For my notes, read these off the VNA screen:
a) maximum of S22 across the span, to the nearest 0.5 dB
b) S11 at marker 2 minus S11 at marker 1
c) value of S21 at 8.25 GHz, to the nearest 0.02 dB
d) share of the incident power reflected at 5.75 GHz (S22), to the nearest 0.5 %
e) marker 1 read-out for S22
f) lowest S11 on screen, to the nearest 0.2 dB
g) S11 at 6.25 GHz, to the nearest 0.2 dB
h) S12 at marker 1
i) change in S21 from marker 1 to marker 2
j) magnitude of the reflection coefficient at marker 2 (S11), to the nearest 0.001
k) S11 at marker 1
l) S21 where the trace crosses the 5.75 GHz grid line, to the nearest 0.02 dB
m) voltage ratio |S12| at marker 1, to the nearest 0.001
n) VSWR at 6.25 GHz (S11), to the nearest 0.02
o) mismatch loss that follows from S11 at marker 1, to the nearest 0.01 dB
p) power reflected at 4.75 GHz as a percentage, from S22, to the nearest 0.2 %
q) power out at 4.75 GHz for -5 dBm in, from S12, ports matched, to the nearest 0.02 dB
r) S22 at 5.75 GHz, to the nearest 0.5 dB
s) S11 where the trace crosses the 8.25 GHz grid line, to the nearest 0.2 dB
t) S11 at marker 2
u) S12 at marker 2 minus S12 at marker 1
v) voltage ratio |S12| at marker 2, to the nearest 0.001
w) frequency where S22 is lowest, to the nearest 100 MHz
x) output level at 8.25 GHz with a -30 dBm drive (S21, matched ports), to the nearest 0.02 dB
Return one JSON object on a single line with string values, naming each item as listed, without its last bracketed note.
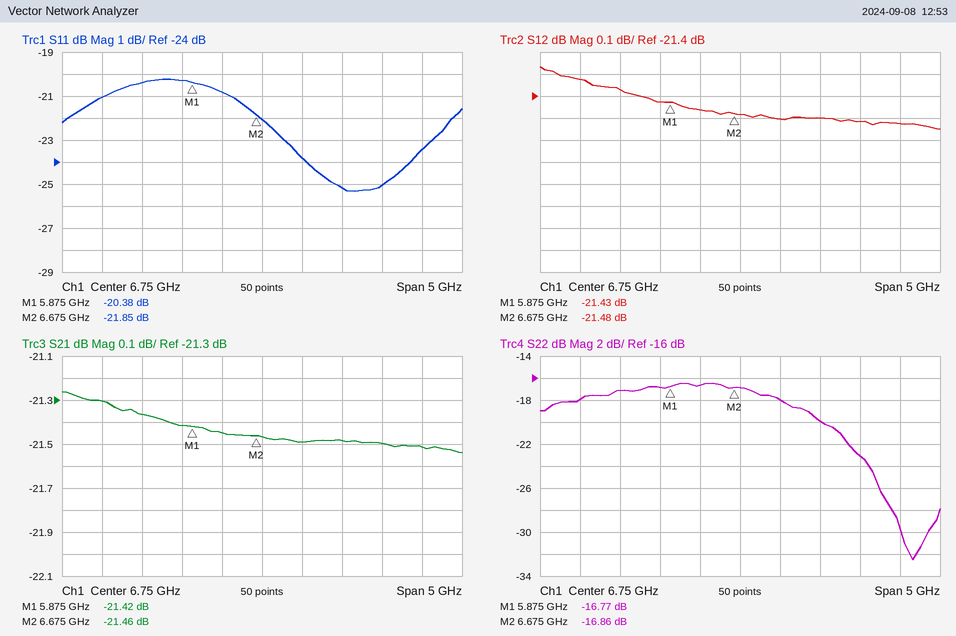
{"maximum of S22 across the span, to the nearest 0.5 dB": "-16.5 dB", "S11 at marker 2 minus S11 at marker 1": "-1.47 dB", "value of S21 at 8.25 GHz, to the nearest 0.02 dB": "-21.50 dB", "share of the incident power reflected at 5.75 GHz (S22), to the nearest 0.5 %": "2.0 %", "marker 1 read-out for S22": "-16.77 dB", "lowest S11 on screen, to the nearest 0.2 dB": "-25.4 dB", "S11 at 6.25 GHz, to the nearest 0.2 dB": "-20.8 dB", "S12 at marker 1": "-21.43 dB", "change in S21 from marker 1 to marker 2": "-0.04 dB", "magnitude of the reflection coefficient at marker 2 (S11), to the nearest 0.001": "0.081", "S11 at marker 1": "-20.38 dB", "S21 where the trace crosses the 5.75 GHz grid line, to the nearest 0.02 dB": "-21.42 dB", "voltage ratio |S12| at marker 1, to the nearest 0.001": "0.085", "VSWR at 6.25 GHz (S11), to the nearest 0.02": "1.20", "mismatch loss that follows from S11 at marker 1, to the nearest 0.01 dB": "0.04 dB", "power reflected at 4.75 GHz as a percentage, from S22, to the nearest 0.2 %": "1.6 %", "power out at 4.75 GHz for -5 dBm in, from S12, ports matched, to the nearest 0.02 dB": "-26.32 dBm", "S22 at 5.75 GHz, to the nearest 0.5 dB": "-17.0 dB", "S11 where the trace crosses the 8.25 GHz grid line, to the nearest 0.2 dB": "-25.0 dB", "S11 at marker 2": "-21.85 dB", "S12 at marker 2 minus S12 at marker 1": "-0.05 dB", "voltage ratio |S12| at marker 2, to the nearest 0.001": "0.084", "frequency where S22 is lowest, to the nearest 100 MHz": "8.9 GHz", "output level at 8.25 GHz with a -30 dBm drive (S21, matched ports), to the nearest 0.02 dB": "-51.50 dBm"}
